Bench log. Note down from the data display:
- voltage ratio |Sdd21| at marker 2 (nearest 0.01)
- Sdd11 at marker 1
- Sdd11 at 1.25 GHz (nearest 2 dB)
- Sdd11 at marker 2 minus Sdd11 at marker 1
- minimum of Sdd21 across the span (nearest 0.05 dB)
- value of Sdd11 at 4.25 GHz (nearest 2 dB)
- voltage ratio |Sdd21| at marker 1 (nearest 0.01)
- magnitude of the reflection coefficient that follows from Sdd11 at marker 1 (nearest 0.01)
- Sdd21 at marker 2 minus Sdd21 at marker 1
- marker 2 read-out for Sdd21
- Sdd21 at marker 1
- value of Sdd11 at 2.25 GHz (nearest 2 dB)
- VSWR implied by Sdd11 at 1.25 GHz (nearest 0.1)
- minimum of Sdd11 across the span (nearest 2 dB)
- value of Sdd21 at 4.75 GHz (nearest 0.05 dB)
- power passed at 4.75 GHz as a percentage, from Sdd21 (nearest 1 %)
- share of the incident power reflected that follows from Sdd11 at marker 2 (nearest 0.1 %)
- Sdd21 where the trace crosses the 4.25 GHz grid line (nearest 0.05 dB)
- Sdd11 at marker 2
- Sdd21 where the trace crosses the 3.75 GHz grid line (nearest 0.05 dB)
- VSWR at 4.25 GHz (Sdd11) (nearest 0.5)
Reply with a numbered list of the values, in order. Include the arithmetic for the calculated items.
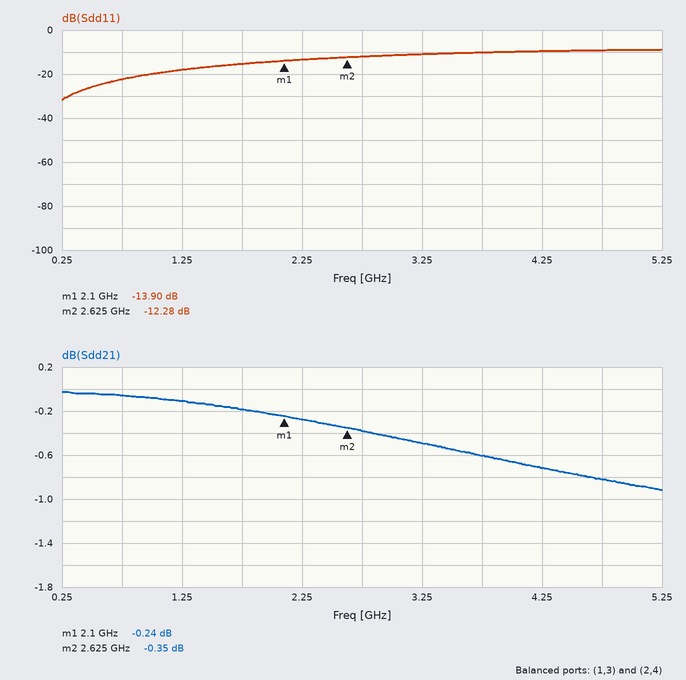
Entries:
1. 10^(-0.35/20) ≈ 0.96
2. -13.90 dB
3. -18 dB
4. -12.28 − (-13.9) = 1.62 dB
5. -0.90 dB
6. -10 dB
7. 10^(-0.24/20) ≈ 0.97
8. 10^(-13.9/20) ≈ 0.20
9. -0.35 − (-0.24) = -0.11 dB
10. -0.35 dB
11. -0.24 dB
12. -14 dB
13. |Γ| = 10^(-18/20) = 0.1259; VSWR = (1 + 0.1259)/(1 − 0.1259) ≈ 1.3
14. -32 dB
15. -0.80 dB
16. 10^(-0.8/10) ≈ 83 %
17. 10^(-12.28/10) ≈ 5.9 %
18. -0.70 dB
19. -12.28 dB
20. -0.60 dB
21. |Γ| = 10^(-10/20) = 0.3162; VSWR = (1 + 0.3162)/(1 − 0.3162) ≈ 1.92, so 2.0 to the nearest 0.5
